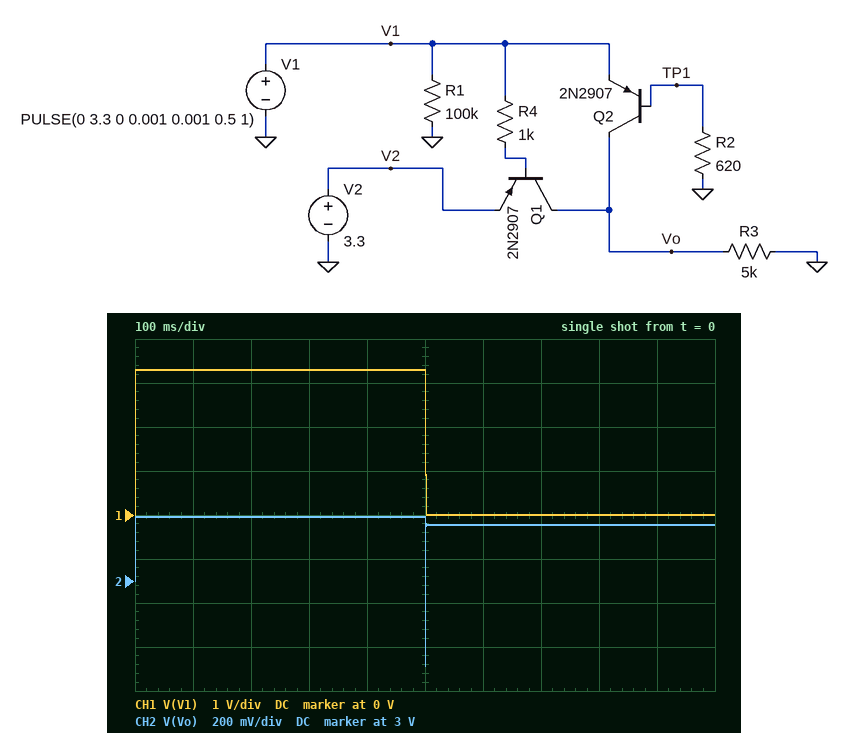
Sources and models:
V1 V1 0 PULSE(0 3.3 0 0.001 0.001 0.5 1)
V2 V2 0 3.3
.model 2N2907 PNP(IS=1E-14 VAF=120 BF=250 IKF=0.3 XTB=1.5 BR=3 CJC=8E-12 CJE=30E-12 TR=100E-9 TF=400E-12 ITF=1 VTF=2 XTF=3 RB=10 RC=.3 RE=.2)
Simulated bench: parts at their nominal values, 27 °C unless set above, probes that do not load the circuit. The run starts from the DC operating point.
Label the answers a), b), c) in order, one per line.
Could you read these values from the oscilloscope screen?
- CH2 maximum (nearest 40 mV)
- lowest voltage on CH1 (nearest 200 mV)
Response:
a) 3.28 V
b) 0 V
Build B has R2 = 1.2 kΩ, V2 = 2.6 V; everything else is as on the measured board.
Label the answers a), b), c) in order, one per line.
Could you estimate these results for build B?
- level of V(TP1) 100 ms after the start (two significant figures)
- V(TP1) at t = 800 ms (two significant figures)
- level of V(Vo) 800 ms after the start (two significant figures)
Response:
a) 2.6 V
b) 1.9 V
c) 2.6 V
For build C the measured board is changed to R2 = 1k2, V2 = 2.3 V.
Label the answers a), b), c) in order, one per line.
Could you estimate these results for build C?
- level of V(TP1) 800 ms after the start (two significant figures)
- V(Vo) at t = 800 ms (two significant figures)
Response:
a) 1.6 V
b) 2.3 V
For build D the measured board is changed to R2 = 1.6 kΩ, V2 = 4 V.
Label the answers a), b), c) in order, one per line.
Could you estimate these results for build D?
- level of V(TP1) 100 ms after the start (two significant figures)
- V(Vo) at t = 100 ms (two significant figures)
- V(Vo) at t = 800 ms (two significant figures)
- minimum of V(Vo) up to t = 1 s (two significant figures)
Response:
a) 2.6 V
b) 3.3 V
c) 4.0 V
d) 3.3 V
